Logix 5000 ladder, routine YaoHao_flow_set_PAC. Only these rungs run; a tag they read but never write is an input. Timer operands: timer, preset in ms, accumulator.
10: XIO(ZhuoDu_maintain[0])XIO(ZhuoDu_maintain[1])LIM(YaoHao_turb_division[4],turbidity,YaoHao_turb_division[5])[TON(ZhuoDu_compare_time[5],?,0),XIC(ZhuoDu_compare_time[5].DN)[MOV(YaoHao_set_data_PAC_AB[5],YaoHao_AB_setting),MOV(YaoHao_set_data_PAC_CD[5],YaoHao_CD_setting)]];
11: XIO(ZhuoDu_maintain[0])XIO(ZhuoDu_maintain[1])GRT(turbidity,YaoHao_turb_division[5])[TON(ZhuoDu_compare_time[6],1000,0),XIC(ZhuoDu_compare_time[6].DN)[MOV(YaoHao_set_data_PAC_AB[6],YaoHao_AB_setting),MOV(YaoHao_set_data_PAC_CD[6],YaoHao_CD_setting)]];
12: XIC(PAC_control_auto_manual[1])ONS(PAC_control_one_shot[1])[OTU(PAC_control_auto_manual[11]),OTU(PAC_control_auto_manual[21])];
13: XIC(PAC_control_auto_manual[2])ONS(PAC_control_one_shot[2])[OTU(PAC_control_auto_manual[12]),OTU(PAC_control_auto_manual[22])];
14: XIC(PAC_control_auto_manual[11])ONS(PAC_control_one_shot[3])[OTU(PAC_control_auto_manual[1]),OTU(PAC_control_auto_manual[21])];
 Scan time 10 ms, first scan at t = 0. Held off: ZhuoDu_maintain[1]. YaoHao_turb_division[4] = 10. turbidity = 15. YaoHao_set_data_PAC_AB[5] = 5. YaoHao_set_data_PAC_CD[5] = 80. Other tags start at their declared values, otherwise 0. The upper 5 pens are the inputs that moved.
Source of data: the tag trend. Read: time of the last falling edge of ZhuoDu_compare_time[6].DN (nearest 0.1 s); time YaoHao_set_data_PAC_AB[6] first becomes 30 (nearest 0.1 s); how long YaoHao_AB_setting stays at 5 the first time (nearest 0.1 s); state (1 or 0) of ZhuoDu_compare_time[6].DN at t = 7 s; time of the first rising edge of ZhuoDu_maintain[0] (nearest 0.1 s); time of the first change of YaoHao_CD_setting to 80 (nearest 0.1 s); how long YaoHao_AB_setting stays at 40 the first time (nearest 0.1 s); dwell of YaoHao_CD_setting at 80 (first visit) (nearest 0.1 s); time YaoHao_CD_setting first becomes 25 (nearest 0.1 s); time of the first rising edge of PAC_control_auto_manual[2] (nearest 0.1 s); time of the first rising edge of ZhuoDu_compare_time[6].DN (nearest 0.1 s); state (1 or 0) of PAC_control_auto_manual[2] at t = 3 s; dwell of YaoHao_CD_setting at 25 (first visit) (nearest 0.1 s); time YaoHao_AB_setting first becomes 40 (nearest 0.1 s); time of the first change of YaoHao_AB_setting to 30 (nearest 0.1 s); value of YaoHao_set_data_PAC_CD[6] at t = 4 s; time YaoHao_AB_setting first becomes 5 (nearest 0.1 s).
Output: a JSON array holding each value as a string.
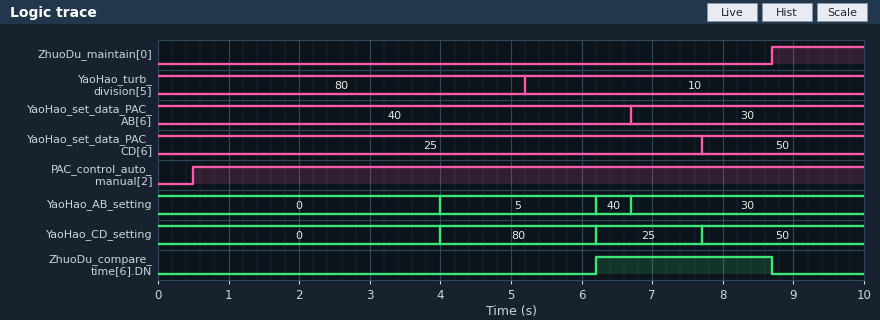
["8.7 s", "6.7 s", "2.2 s", "1", "8.7 s", "4.0 s", "0.5 s", "2.2 s", "6.2 s", "0.5 s", "6.2 s", "1", "1.5 s", "6.2 s", "6.7 s", "25", "4.0 s"]
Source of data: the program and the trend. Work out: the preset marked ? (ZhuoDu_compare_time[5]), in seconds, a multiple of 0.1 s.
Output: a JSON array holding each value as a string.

["4.0 s"]
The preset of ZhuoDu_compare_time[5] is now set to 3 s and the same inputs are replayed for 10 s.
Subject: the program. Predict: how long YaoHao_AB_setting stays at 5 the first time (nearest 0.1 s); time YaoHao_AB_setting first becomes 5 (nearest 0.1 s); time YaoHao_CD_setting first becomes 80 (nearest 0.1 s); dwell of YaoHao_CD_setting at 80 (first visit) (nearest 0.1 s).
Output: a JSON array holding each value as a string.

["3.2 s", "3.0 s", "3.0 s", "3.2 s"]
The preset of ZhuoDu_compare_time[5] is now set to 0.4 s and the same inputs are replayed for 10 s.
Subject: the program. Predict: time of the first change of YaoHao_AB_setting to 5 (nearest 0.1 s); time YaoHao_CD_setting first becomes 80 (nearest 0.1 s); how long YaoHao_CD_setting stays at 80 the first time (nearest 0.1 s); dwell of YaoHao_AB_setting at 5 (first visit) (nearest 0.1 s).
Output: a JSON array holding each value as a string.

["0.4 s", "0.4 s", "5.8 s", "5.8 s"]
